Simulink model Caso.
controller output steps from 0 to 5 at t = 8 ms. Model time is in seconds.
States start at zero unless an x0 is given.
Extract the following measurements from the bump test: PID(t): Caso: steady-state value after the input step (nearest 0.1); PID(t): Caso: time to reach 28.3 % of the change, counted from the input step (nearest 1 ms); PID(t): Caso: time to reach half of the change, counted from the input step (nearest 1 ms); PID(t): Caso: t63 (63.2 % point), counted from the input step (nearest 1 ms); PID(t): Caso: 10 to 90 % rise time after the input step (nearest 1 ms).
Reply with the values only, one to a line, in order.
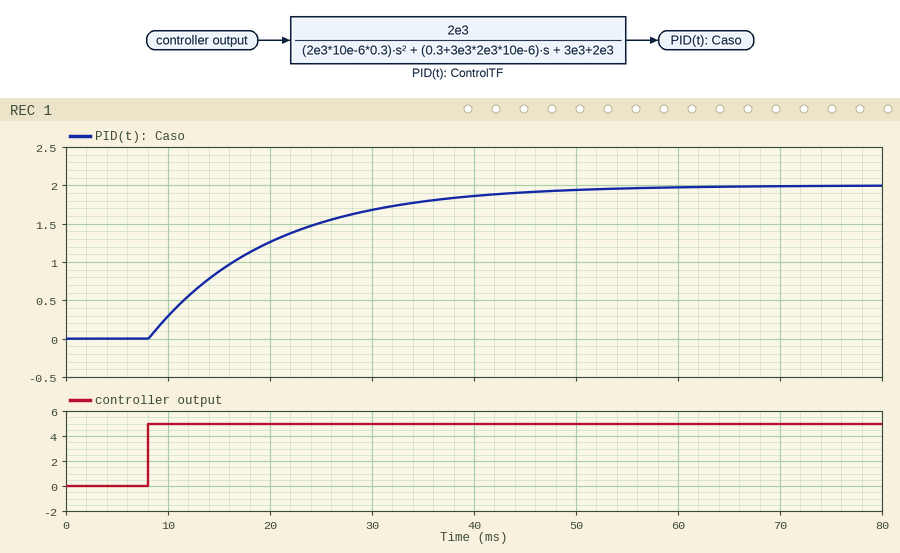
2.0
4 ms
8 ms
12 ms
26 ms
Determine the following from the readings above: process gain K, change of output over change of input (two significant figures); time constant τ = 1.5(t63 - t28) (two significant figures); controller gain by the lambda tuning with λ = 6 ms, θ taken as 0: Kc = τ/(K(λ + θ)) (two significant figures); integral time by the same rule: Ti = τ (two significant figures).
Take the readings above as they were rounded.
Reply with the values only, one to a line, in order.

0.40
12 ms
5.0
12 ms
